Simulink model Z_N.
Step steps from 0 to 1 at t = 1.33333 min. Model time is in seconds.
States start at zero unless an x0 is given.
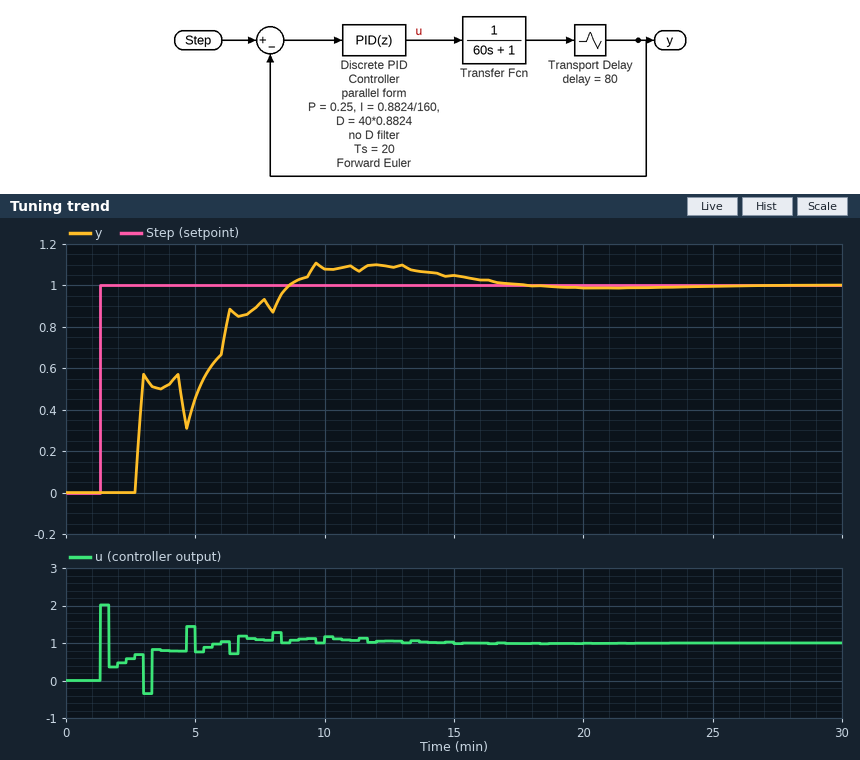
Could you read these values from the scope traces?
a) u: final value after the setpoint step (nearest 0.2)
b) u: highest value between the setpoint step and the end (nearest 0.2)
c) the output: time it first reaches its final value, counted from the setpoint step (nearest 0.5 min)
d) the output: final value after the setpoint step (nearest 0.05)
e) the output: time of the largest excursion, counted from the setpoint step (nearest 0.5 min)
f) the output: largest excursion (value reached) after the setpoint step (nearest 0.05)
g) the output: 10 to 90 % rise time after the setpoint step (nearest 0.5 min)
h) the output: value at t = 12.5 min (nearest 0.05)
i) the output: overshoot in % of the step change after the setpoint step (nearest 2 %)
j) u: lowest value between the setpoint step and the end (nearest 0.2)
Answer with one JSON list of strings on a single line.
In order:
["1.0", "2.0", "7.5 min", "1.00", "8.5 min", "1.10", "4.5 min", "1.10", "10 %", "-0.4"]
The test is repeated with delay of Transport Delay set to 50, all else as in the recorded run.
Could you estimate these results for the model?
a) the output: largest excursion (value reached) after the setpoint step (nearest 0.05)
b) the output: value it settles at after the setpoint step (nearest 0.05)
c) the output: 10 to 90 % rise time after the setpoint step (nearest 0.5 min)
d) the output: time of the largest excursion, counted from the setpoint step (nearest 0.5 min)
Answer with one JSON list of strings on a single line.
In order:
["1.05", "1.00", "5.5 min", "10.5 min"]
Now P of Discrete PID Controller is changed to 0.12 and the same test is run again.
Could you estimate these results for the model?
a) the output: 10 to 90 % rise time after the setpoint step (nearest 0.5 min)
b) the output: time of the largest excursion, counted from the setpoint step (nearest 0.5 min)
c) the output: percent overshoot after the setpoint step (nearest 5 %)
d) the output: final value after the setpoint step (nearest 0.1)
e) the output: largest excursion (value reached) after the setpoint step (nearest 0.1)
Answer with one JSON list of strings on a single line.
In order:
["5.0 min", "10.5 min", "15 %", "1.0", "1.2"]
